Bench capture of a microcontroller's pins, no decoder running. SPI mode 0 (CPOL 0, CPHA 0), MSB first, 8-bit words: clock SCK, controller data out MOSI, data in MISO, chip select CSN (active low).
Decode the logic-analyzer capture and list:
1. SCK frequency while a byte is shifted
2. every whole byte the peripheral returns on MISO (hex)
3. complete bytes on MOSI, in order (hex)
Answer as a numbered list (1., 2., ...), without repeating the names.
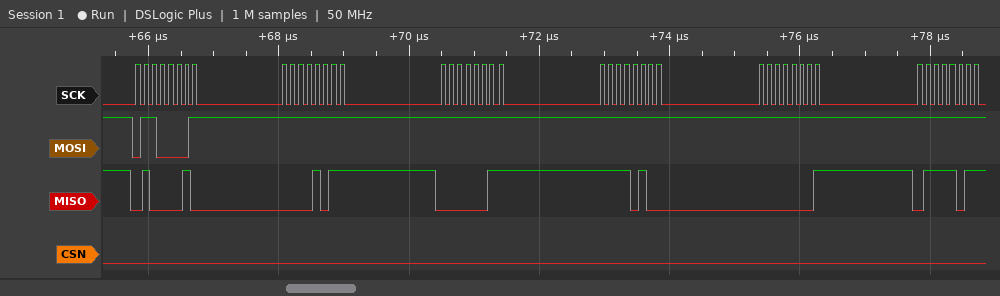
1. 8 MHz
2. 42 0B 03 F4 01 7B
3. 61 FF FF FF FF FF
